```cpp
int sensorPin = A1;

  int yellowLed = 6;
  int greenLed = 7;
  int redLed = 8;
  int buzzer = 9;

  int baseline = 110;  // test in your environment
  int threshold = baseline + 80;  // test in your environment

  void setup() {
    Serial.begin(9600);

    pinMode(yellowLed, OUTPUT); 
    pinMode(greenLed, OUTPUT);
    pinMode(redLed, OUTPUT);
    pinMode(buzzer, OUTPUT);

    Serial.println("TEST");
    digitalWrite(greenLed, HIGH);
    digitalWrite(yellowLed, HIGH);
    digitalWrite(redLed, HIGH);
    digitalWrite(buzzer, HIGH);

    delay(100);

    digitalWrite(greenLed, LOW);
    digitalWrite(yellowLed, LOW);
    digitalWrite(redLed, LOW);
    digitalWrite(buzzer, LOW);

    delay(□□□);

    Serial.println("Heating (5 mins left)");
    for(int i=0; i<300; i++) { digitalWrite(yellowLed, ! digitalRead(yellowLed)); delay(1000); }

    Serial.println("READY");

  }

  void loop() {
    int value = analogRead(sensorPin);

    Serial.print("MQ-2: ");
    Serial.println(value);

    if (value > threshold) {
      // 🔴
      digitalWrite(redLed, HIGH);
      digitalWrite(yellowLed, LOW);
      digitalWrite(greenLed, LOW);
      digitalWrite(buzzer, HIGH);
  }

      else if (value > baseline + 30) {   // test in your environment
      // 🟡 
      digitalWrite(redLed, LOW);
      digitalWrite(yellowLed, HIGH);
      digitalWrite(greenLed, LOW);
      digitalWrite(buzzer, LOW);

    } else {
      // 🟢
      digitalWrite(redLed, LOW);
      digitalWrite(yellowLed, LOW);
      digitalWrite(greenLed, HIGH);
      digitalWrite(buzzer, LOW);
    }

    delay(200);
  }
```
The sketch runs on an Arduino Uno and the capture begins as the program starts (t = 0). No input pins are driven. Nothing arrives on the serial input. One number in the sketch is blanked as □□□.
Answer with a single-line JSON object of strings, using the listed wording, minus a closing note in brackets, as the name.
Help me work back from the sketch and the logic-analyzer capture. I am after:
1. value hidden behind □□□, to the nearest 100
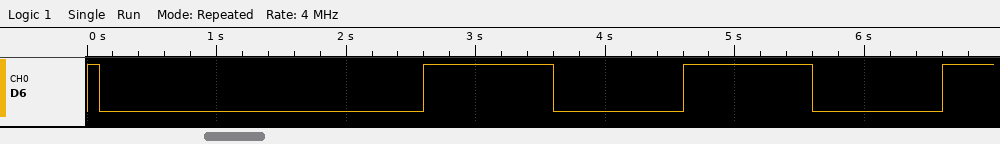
{"value hidden behind □□□, to the nearest 100": "2500"}
